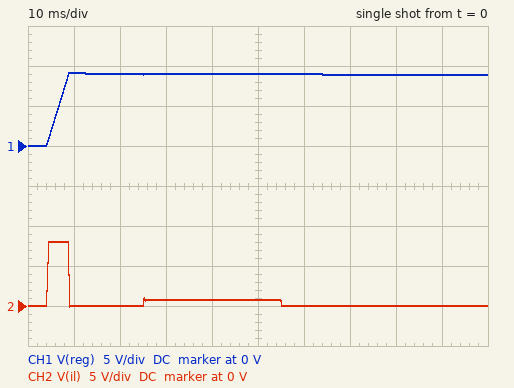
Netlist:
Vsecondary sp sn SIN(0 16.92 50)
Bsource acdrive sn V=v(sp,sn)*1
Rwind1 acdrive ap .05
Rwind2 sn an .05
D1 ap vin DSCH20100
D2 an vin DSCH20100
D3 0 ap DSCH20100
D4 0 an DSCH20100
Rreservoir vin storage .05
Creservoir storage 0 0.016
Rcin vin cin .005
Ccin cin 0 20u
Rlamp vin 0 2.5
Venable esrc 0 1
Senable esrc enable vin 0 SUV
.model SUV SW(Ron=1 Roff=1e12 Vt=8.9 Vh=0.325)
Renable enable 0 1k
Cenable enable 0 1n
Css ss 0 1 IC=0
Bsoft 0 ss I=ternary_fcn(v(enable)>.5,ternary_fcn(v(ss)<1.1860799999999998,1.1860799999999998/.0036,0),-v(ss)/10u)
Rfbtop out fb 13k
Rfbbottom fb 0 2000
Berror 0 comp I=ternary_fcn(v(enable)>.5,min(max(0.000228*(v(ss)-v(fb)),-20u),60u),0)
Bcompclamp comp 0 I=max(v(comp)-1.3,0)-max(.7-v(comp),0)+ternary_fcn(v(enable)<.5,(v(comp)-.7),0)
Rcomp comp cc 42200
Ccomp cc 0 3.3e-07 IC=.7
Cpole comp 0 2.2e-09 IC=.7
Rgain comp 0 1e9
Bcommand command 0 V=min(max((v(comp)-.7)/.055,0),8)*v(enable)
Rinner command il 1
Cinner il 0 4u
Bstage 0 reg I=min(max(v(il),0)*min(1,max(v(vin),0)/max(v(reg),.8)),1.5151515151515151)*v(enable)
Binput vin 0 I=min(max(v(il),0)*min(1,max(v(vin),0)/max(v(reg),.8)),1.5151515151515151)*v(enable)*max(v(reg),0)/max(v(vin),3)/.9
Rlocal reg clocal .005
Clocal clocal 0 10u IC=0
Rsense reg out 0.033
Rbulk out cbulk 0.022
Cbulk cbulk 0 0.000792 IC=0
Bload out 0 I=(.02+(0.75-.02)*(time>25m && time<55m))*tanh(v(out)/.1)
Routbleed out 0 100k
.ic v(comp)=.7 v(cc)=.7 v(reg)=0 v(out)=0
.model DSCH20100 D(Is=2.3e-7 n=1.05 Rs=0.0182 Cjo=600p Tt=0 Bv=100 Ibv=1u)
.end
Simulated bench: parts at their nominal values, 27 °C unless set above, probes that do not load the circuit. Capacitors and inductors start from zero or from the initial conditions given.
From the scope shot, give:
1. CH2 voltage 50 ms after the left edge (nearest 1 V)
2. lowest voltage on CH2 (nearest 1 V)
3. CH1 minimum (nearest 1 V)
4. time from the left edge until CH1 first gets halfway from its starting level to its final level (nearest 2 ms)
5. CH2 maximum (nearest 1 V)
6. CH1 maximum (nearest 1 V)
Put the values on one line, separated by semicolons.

1 V; 0 V; 0 V; 6 ms; 8 V; 9 V
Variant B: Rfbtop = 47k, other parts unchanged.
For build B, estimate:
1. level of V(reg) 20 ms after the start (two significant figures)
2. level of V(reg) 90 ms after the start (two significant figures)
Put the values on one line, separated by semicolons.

30 V; 29 V
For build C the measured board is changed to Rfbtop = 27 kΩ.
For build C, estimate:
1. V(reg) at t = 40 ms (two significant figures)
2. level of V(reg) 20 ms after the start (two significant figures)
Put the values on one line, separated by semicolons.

17 V; 18 V
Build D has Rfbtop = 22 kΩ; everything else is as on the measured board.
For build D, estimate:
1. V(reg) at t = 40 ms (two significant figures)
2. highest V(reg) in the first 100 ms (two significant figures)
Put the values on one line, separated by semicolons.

14 V; 15 V
